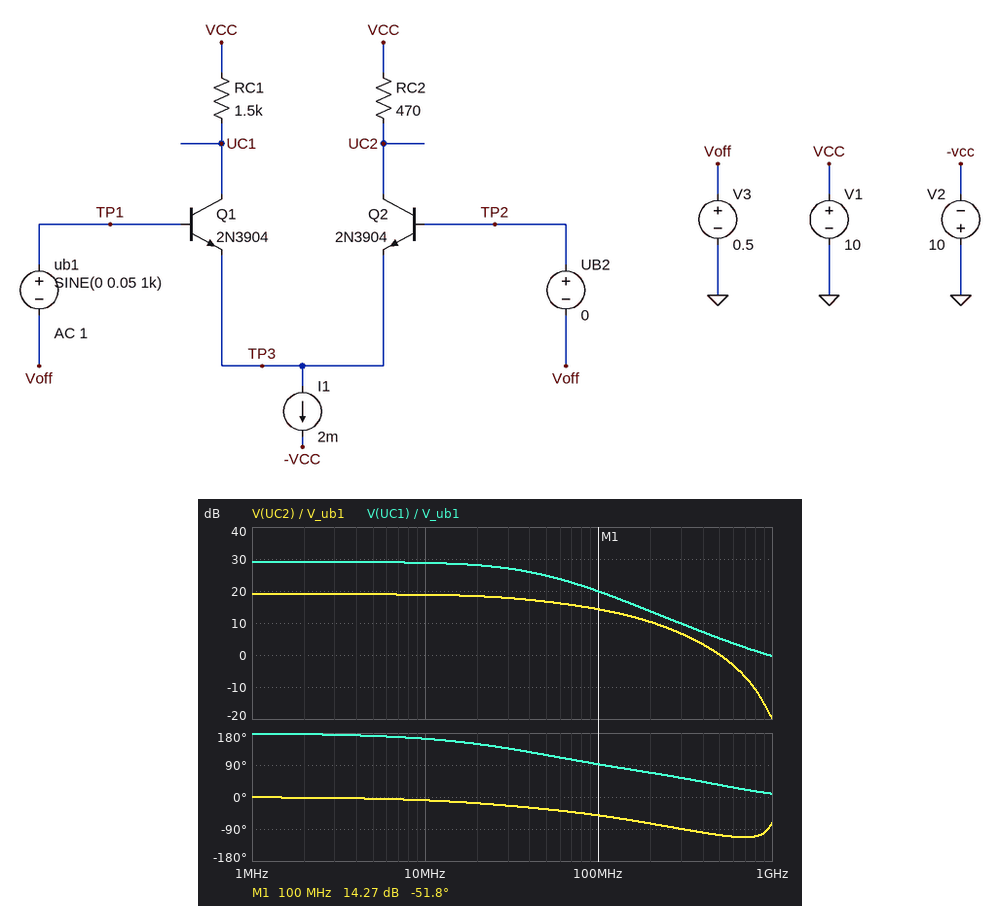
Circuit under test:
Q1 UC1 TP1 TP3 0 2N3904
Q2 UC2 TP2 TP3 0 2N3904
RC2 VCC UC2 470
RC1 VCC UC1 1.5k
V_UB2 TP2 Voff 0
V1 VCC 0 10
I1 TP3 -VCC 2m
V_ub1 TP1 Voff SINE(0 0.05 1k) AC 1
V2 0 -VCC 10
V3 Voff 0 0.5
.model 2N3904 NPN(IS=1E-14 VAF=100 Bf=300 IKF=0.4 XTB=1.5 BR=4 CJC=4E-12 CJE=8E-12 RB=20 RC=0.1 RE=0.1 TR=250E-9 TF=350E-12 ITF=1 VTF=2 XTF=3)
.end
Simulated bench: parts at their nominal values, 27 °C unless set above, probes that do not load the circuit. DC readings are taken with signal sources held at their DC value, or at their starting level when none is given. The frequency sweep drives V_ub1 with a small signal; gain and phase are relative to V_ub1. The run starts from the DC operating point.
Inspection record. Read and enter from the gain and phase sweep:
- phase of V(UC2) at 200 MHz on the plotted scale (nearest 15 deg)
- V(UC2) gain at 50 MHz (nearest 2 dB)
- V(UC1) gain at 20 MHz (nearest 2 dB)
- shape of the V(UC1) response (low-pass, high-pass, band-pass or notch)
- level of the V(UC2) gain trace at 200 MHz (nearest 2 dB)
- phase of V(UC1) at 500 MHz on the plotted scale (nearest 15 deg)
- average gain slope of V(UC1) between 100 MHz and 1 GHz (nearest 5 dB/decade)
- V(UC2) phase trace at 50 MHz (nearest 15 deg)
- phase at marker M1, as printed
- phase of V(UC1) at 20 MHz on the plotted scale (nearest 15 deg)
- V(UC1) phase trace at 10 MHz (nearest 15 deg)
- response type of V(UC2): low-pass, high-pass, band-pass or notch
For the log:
-75 deg
16 dB
28 dB
low-pass
10 dB
30 deg
-20 dB/decade
-30 deg
-51.8 deg
150 deg
165 deg
low-pass
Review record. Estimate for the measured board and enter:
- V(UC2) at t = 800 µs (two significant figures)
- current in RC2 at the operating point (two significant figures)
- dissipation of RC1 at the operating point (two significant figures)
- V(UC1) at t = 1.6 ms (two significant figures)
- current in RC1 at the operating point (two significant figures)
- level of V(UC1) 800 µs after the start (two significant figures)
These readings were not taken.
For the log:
9.2 V
1.0 mA
1.5 mW
9.3 V
990 µA
9.6 V
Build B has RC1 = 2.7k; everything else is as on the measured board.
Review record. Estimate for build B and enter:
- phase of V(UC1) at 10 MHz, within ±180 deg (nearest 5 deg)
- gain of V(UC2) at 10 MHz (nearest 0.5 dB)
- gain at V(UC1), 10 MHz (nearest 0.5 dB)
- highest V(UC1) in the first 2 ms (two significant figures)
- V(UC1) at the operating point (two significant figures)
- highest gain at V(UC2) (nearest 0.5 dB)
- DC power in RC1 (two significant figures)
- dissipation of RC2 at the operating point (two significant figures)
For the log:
155 deg
18.5 dB
33.5 dB
9.3 V
7.3 V
19.0 dB
2.6 mW
480 µW
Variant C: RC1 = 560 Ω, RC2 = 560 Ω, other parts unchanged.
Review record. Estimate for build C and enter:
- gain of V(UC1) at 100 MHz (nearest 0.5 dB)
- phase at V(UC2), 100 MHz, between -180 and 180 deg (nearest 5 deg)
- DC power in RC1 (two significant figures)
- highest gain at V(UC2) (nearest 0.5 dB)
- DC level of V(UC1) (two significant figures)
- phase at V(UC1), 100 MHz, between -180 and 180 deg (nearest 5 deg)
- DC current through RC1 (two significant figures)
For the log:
16.5 dB
-60 deg
560 µW
20.5 dB
9.4 V
115 deg
1.0 mA
